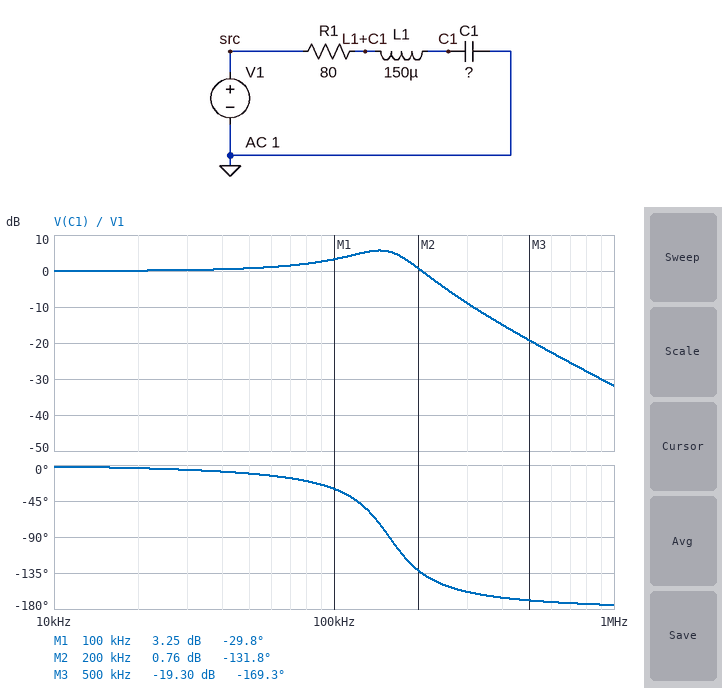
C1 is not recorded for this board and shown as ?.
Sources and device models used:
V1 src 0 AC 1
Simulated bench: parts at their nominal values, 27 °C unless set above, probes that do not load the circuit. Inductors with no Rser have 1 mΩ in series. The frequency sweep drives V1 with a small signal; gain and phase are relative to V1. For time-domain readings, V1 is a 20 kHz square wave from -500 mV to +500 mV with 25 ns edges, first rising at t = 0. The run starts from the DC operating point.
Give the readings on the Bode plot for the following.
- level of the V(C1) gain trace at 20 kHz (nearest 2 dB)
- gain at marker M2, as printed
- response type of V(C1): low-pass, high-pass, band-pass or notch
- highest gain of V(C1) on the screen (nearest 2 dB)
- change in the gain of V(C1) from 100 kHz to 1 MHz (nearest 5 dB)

0 dB
0.76 dB
low-pass
6 dB
-35 dB
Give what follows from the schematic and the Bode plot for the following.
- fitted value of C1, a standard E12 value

6.8 nF
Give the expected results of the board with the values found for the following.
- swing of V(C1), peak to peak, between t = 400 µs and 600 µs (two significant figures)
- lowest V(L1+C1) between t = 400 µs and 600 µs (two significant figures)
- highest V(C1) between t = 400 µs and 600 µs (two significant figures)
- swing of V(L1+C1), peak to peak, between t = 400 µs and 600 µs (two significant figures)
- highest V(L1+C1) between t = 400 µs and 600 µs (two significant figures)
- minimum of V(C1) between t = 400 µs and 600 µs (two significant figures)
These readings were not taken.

1.8 V
-660 mV
920 mV
1.3 V
660 mV
-920 mV
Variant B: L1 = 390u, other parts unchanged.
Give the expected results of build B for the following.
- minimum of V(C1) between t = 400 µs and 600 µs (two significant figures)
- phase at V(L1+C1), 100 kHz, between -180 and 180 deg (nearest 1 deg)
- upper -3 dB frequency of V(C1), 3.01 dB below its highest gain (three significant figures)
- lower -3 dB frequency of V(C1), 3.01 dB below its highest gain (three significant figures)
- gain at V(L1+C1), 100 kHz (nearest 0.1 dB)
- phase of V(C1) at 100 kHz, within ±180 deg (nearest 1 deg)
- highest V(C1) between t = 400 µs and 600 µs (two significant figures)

-1.1 V
82 deg
110 kHz
76.6 kHz
-17.3 dB
-98 deg
1.1 V
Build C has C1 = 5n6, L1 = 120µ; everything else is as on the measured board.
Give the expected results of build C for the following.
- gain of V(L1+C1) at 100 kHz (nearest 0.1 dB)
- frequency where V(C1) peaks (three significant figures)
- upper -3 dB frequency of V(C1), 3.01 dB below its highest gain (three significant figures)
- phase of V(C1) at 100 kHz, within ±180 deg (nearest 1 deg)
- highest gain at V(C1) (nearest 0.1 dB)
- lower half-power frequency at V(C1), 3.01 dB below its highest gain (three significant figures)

-0.6 dB
179 kHz
228 kHz
-21 deg
5.6 dB
111 kHz
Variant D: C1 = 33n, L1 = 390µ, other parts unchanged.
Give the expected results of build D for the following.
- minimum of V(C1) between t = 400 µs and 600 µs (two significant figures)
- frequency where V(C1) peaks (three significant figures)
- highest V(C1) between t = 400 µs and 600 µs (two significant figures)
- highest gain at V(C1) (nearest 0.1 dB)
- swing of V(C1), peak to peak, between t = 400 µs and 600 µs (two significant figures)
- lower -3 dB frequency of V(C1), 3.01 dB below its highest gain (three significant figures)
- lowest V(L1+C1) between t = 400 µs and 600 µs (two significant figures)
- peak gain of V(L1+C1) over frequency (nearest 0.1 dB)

-770 mV
37.9 kHz
770 mV
3.3 dB
1.5 V
9.41 kHz
-620 mV
0 dB
